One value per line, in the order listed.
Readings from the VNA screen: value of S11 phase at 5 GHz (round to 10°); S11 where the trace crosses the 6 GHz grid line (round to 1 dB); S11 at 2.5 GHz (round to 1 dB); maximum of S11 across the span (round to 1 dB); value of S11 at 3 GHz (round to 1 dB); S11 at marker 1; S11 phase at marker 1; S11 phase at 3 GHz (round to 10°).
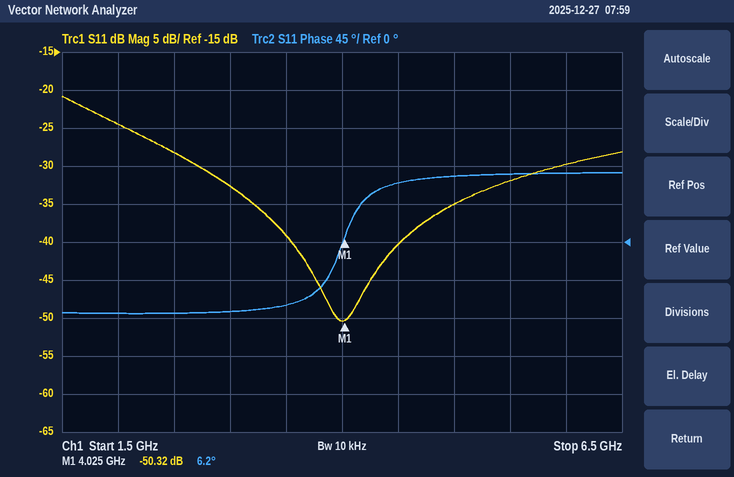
80°
-30 dB
-28 dB
-21 dB
-33 dB
-50.32 dB
6.2°
-80°
